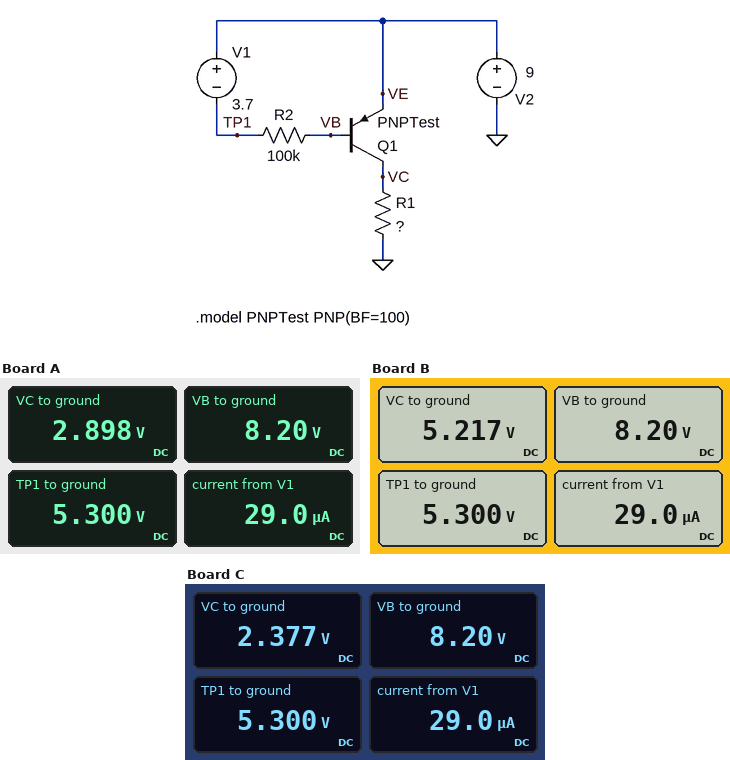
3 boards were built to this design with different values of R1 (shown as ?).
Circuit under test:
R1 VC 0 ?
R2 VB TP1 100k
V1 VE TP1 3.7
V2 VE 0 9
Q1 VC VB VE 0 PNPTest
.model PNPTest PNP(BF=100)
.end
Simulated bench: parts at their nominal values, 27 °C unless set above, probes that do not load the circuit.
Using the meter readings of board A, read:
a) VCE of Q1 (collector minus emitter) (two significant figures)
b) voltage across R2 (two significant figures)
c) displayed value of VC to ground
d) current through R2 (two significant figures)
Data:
-6.1 V
2.9 V
2.898 V
29 µA
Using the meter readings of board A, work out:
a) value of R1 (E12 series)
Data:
1 kΩ
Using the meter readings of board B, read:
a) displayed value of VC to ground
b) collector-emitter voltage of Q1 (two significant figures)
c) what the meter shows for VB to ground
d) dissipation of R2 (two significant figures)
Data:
5.217 V
-3.8 V
8.20 V
84 µW
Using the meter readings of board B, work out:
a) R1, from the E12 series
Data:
1.8 kΩ
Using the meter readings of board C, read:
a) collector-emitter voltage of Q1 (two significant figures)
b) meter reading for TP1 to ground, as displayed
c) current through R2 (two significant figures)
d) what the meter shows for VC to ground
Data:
-6.6 V
5.300 V
29 µA
2.377 V
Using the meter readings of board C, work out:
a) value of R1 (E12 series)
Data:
820 Ω
